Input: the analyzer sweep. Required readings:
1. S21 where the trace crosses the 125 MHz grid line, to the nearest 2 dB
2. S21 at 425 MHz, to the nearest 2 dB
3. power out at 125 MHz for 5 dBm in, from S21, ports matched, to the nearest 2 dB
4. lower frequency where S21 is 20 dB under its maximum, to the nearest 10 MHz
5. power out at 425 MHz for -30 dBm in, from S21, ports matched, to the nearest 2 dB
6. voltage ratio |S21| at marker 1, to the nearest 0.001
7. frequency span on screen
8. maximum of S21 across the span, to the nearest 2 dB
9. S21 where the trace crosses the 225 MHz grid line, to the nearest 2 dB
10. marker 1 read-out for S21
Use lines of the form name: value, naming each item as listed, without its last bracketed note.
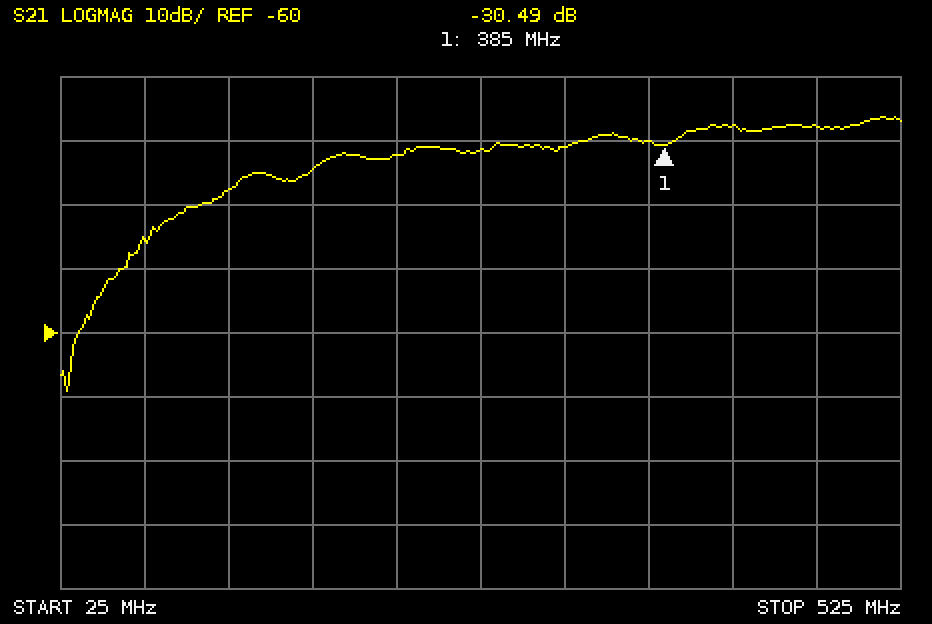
S21 where the trace crosses the 125 MHz grid line, to the nearest 2 dB: -38 dB
S21 at 425 MHz, to the nearest 2 dB: -28 dB
power out at 125 MHz for 5 dBm in, from S21, ports matched, to the nearest 2 dB: -32 dBm
lower frequency where S21 is 20 dB under its maximum, to the nearest 10 MHz: 70 MHz
power out at 425 MHz for -30 dBm in, from S21, ports matched, to the nearest 2 dB: -58 dBm
voltage ratio |S21| at marker 1, to the nearest 0.001: 0.030
frequency span on screen: 500 MHz
maximum of S21 across the span, to the nearest 2 dB: -26 dB
S21 where the trace crosses the 225 MHz grid line, to the nearest 2 dB: -32 dB
marker 1 read-out for S21: -30.49 dB
